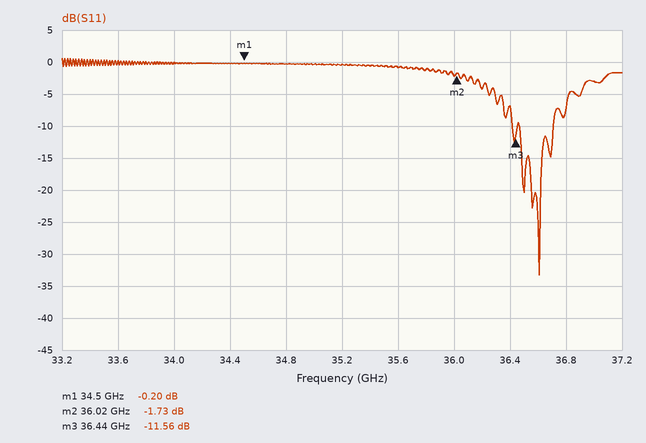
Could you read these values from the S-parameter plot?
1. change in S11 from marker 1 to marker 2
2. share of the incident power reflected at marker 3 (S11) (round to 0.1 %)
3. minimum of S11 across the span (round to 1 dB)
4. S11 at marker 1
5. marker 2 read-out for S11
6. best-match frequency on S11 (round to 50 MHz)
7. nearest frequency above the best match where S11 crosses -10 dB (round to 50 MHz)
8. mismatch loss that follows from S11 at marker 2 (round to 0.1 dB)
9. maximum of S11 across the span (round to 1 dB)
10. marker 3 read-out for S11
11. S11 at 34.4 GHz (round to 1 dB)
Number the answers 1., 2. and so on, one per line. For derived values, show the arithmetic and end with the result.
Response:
1. -1.73 − (-0.2) = -1.53 dB
2. 10^(-11.56/10) ≈ 7.0 %
3. -33 dB
4. -0.20 dB
5. -1.73 dB
6. 36.60 GHz
7. 36.70 GHz
8. −10 log10(1 − 10^(-1.73/10)) ≈ 4.8 dB
9. 1 dB
10. -11.56 dB
11. 0 dB
